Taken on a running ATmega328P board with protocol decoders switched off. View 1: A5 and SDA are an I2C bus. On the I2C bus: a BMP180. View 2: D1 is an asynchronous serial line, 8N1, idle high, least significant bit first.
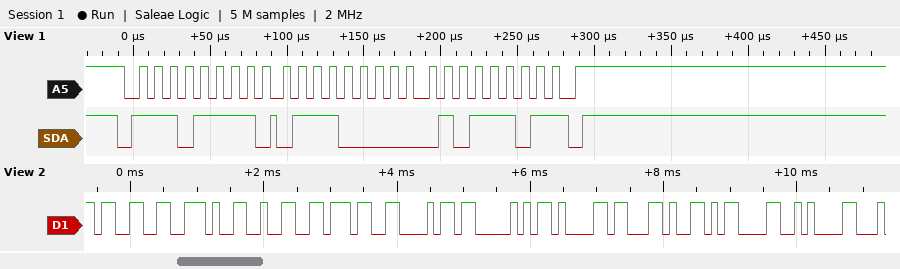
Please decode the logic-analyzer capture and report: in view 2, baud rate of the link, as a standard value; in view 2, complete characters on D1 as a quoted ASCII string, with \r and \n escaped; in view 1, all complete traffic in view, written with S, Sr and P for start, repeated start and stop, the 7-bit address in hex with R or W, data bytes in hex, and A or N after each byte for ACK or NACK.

9600 baud
"3.27hPa,\r\n"
S 77R A 70 A 5D N P
